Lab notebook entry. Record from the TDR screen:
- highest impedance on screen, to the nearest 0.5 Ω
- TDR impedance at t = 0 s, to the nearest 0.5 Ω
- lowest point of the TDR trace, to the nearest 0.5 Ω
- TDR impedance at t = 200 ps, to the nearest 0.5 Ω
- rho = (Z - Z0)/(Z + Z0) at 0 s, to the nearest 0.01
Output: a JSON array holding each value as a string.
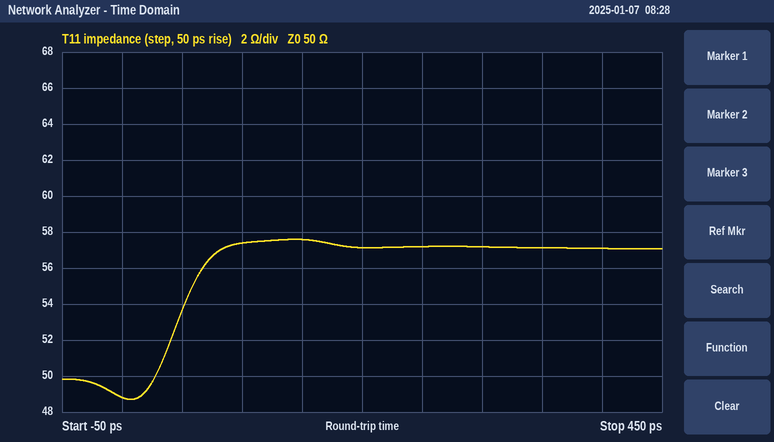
["57.5 Ω", "49.0 Ω", "48.5 Ω", "57.0 Ω", "-0.01"]
